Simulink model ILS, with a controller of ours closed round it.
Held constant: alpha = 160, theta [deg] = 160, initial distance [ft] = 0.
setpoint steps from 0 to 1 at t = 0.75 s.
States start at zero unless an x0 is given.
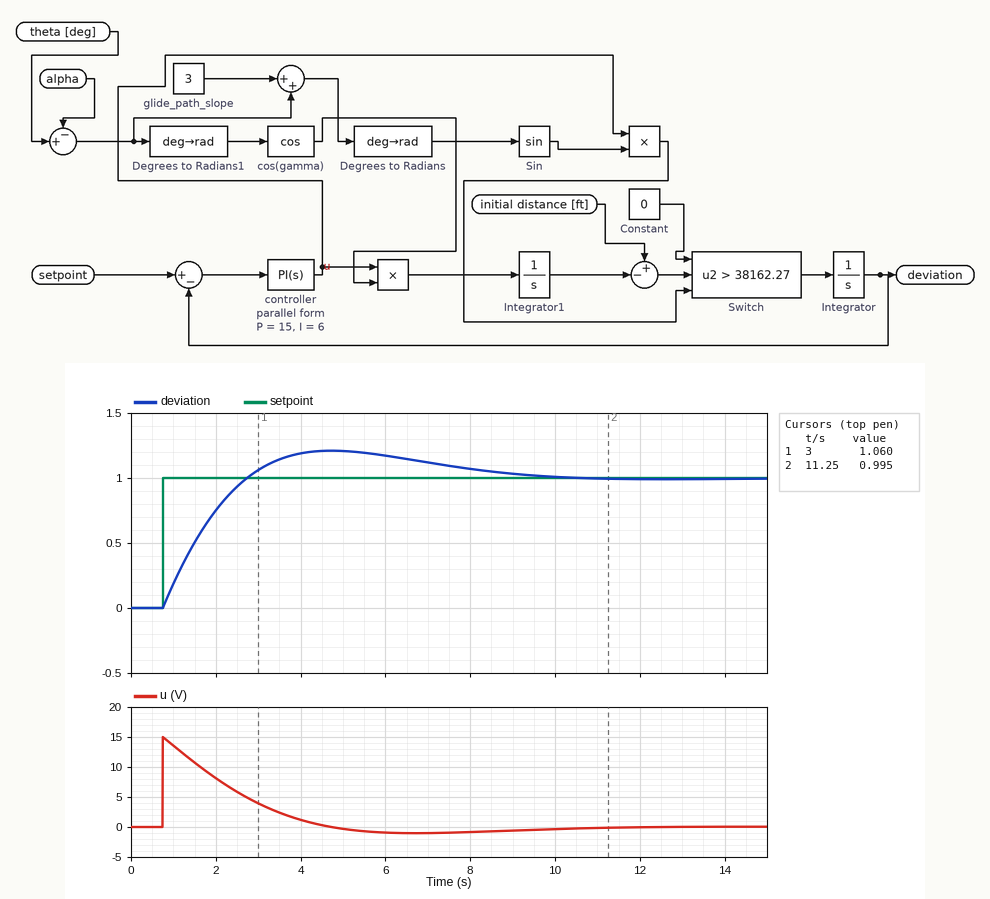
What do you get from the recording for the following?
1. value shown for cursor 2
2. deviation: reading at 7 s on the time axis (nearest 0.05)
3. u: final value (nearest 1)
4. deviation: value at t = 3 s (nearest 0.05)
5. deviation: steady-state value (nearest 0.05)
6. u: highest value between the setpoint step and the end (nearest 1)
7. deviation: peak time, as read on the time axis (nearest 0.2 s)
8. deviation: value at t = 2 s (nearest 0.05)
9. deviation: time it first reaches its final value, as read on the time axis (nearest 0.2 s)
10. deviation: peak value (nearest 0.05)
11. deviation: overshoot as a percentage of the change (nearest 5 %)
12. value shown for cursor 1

0.995
1.10
0
1.05
1.00
15
4.8 s
0.75
2.8 s
1.20
20 %
1.060
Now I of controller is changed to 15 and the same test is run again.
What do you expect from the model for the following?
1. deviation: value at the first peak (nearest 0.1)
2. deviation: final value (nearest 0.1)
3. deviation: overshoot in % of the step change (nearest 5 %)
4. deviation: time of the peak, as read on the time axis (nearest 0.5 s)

1.3
1.0
35 %
3.5 s
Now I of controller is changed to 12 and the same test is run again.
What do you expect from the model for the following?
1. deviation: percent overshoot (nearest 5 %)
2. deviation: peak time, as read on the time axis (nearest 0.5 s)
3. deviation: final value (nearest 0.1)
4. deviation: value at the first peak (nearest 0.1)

30 %
4.0 s
1.0
1.3
